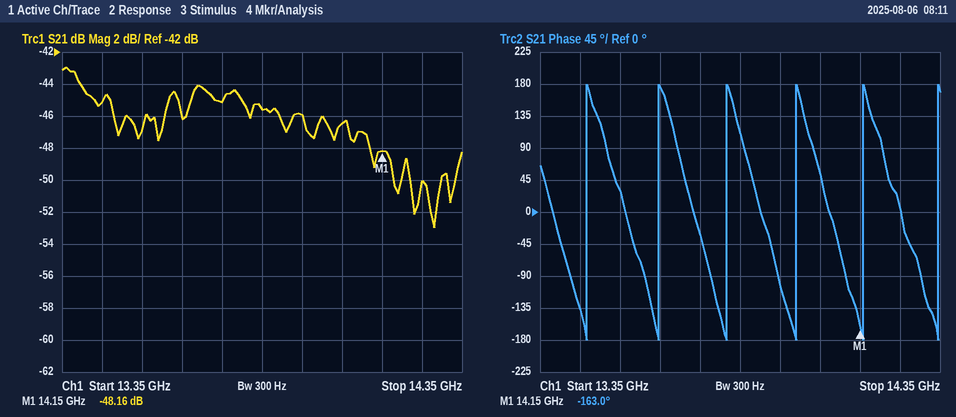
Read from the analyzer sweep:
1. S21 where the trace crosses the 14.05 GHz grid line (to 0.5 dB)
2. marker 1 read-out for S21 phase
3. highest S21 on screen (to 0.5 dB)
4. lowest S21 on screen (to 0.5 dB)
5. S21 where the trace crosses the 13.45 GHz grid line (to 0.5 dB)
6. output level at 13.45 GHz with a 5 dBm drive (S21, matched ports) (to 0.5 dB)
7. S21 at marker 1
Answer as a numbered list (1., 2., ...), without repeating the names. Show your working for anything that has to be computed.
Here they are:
1. -46.5 dB
2. -163.0°
3. -43.0 dB
4. -53.0 dB
5. -45.0 dB
6. 5 dBm + (-45.0 dB) = -40.0 dBm
7. -48.16 dB
